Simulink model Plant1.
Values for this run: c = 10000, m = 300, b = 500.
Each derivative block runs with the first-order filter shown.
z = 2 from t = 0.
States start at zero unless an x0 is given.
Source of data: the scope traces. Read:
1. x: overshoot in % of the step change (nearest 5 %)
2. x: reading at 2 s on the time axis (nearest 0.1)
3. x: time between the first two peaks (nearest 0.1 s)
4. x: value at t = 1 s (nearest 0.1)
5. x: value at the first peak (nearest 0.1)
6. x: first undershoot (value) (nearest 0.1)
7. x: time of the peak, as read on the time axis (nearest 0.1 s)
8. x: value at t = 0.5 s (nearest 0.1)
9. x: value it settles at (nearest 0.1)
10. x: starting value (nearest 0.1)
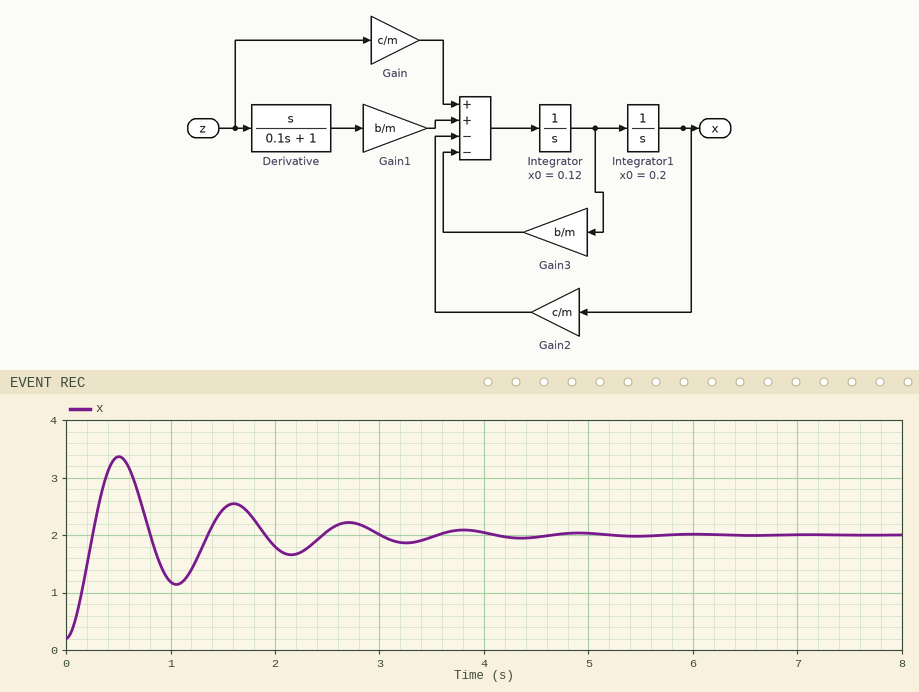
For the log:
75 %
1.8
1.1 s
1.2
3.4
1.1
0.5 s
3.4
2.0
0.2
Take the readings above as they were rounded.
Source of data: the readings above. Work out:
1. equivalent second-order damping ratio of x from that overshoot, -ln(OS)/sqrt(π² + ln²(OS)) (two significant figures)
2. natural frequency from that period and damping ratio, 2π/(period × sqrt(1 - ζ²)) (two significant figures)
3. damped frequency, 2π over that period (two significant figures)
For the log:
0.091
5.7 rad/s
5.7 rad/s
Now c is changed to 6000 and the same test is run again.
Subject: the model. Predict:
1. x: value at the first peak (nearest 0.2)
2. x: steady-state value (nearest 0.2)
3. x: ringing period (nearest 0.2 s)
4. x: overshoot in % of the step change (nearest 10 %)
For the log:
3.2
2.0
1.4 s
70 %
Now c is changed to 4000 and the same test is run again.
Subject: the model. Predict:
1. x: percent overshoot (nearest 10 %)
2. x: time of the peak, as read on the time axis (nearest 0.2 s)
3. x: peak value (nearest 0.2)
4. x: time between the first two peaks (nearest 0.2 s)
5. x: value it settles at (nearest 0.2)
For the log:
60 %
0.8 s
3.2
1.8 s
2.0
